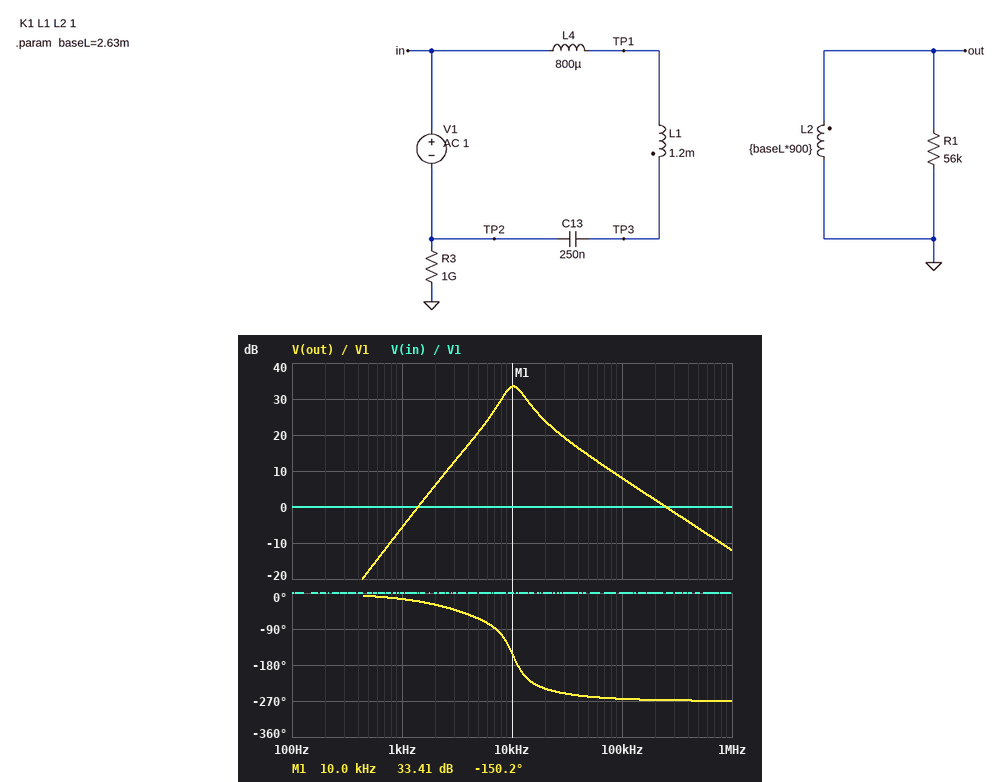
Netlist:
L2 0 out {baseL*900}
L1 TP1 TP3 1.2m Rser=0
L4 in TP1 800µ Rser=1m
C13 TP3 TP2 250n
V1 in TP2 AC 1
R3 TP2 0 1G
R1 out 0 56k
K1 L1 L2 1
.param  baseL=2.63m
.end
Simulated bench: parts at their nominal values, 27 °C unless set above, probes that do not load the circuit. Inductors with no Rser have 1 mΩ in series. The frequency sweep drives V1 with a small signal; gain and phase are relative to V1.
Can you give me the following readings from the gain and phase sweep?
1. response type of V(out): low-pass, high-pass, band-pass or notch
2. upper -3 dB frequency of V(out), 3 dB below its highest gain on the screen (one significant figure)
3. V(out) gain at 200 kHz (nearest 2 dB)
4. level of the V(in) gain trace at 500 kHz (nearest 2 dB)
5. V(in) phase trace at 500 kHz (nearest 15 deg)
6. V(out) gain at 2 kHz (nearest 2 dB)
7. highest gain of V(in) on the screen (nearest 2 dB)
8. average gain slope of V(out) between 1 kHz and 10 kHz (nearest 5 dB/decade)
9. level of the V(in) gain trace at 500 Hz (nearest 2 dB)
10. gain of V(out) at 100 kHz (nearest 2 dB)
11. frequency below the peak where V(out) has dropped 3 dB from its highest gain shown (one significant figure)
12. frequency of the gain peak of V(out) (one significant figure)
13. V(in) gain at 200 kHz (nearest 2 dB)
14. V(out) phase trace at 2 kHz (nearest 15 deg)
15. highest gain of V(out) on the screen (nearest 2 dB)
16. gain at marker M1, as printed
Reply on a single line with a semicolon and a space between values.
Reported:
band-pass; 10 kHz; 2 dB; 0 dB; 0 deg; 6 dB; 0 dB; 40 dB/decade; 0 dB; 8 dB; 8 kHz; 10 kHz; 0 dB; -30 deg; 34 dB; 33.41 dB
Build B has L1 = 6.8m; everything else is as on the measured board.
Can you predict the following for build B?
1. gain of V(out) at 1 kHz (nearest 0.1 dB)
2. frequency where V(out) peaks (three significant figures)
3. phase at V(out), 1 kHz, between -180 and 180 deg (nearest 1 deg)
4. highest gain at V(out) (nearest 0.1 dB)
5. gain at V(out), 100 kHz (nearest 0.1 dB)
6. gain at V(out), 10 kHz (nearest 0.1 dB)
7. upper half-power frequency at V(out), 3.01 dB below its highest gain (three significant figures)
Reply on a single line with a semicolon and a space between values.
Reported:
2.3 dB; 4.94 kHz; -16 deg; 27.1 dB; 15.1 dB; 25.7 dB; 20.0 kHz
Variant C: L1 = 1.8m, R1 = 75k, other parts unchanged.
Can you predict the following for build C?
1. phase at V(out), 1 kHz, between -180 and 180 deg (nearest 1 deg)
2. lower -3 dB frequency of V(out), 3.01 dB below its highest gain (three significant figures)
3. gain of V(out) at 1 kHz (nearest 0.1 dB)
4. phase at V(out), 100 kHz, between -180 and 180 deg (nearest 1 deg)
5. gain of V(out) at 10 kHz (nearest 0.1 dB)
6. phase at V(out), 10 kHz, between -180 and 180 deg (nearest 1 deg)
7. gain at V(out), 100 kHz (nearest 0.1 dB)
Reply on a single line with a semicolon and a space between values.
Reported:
-11 deg; 6.26 kHz; -3.8 dB; 99 deg; 32.0 dB; -165 deg; 12.3 dB
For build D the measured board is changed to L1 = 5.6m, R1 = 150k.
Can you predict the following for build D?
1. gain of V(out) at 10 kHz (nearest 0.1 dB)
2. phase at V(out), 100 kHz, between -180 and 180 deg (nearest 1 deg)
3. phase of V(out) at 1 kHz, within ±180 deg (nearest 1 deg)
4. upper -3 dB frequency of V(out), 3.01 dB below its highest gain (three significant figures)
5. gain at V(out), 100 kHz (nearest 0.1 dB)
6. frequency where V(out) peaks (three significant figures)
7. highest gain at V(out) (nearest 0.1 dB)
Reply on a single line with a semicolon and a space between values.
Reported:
26.6 dB; 129 deg; -6 deg; 5.19 kHz; 21.1 dB; 4.14 kHz; 34.6 dB
